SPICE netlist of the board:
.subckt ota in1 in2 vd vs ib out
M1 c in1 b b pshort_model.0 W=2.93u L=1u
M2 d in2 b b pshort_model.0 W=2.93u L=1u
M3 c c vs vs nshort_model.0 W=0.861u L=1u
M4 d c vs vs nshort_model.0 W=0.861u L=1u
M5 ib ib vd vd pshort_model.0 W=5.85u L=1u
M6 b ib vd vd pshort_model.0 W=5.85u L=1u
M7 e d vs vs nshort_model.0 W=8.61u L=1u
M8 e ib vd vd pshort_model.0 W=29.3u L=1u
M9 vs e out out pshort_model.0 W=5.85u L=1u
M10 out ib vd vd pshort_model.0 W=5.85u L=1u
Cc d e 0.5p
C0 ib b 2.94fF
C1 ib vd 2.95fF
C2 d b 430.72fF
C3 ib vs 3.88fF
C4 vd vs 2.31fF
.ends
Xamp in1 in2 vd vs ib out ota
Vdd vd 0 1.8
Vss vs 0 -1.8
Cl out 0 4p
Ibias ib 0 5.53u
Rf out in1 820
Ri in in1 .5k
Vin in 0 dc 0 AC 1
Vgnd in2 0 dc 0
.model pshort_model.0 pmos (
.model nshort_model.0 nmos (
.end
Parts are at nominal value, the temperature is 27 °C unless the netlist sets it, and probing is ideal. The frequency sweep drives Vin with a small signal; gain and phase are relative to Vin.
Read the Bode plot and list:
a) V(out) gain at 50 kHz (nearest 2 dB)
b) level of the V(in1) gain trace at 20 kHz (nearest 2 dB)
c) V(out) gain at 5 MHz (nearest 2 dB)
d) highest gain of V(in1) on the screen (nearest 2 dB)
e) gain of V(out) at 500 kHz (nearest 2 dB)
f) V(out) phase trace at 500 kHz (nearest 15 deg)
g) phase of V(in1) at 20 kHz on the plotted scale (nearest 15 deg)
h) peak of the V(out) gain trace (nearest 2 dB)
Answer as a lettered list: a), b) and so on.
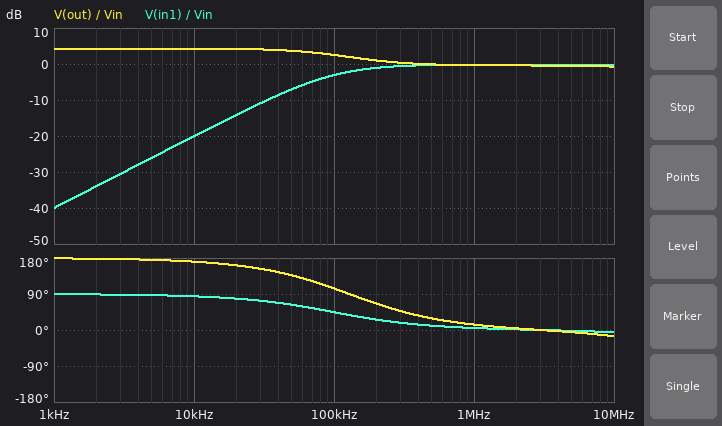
a) 4 dB
b) -14 dB
c) 0 dB
d) 0 dB
e) 0 dB
f) 30 deg
g) 75 deg
h) 4 dB
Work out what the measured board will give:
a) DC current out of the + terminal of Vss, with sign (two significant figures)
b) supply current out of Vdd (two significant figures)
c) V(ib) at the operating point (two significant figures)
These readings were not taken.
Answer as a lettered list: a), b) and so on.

a) -39 µA
b) 44 µA
c) 1.5 V
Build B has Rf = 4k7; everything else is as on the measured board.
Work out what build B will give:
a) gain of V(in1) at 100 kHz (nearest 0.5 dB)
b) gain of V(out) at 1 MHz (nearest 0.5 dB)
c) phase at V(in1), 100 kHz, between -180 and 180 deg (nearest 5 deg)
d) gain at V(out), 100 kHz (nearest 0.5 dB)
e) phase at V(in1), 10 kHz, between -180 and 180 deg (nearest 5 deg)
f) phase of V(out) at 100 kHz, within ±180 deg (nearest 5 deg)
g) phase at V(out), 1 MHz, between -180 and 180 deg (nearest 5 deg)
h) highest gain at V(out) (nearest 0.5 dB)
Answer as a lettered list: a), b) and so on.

a) -2.5 dB
b) 1.5 dB
c) 40 deg
d) 16.0 dB
e) 85 deg
f) 125 deg
g) 45 deg
h) 19.5 dB
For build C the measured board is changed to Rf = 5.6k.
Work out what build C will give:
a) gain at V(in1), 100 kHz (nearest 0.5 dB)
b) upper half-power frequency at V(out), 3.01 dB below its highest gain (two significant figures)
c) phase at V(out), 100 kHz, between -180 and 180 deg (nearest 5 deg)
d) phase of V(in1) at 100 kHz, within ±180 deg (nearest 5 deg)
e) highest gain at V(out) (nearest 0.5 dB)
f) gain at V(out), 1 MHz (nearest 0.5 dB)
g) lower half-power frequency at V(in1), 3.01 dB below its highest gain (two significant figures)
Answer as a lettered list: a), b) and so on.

a) -2.5 dB
b) 86 kHz
c) 125 deg
d) 40 deg
e) 21.0 dB
f) 2.0 dB
g) 85 kHz
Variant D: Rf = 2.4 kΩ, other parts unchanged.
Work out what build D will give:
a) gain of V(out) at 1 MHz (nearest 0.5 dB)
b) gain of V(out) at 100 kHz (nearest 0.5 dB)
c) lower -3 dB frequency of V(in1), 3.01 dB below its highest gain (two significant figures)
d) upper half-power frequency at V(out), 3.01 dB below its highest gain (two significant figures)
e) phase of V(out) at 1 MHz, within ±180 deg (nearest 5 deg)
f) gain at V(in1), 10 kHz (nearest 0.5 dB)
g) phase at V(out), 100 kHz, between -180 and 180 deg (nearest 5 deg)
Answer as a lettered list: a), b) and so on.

a) 0 dB
b) 10.5 dB
c) 93 kHz
d) 97 kHz
e) 30 deg
f) -19.5 dB
g) 120 deg
